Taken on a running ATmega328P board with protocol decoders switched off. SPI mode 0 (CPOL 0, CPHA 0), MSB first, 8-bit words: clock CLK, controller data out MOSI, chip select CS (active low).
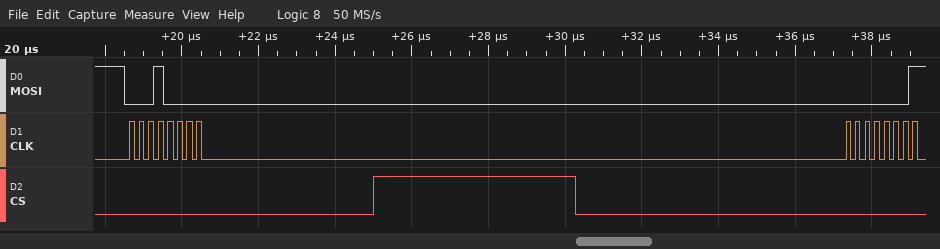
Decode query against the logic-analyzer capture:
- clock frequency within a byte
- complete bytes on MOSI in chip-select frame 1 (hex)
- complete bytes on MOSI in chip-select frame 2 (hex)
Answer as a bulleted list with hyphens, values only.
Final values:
- 4 MHz
- 10
- 01
